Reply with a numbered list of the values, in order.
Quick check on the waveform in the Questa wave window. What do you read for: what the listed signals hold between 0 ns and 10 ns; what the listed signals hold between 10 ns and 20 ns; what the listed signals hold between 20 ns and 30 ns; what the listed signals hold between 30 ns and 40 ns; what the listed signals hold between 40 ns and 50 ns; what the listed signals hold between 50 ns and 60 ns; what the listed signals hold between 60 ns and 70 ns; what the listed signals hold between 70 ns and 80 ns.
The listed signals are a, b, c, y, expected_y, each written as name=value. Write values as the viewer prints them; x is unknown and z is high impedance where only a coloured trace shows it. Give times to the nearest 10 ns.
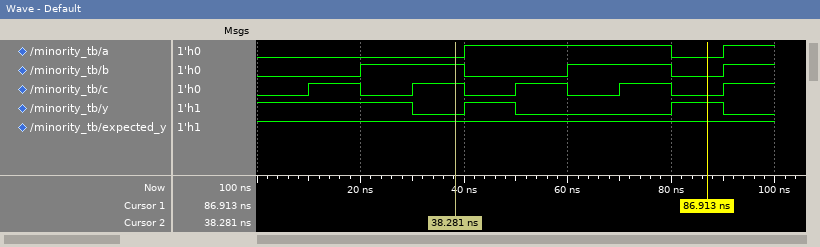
1. a=0, b=0, c=0, y=1, expected_y=1
2. a=0, b=0, c=1, y=1, expected_y=1
3. a=0, b=1, c=0, y=1, expected_y=1
4. a=0, b=1, c=1, y=0, expected_y=1
5. a=1, b=0, c=0, y=1, expected_y=1
6. a=1, b=0, c=1, y=0, expected_y=1
7. a=1, b=1, c=0, y=0, expected_y=1
8. a=1, b=1, c=1, y=0, expected_y=1
